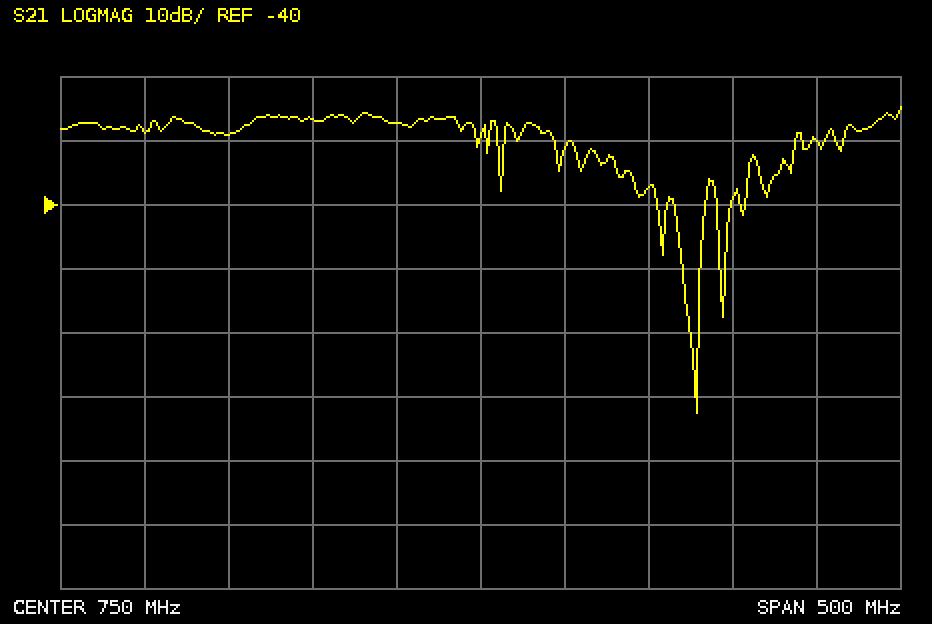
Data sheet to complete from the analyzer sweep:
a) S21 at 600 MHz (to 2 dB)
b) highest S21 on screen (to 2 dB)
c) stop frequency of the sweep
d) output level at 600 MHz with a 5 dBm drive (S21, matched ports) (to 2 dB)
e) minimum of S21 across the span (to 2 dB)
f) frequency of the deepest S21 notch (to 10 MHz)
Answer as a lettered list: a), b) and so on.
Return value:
a) -30 dB
b) -24 dB
c) 1 GHz
d) -24 dBm
e) -72 dB
f) 880 MHz
